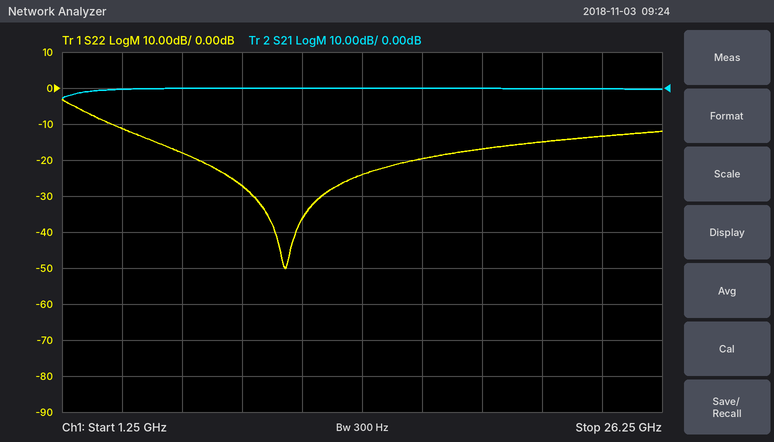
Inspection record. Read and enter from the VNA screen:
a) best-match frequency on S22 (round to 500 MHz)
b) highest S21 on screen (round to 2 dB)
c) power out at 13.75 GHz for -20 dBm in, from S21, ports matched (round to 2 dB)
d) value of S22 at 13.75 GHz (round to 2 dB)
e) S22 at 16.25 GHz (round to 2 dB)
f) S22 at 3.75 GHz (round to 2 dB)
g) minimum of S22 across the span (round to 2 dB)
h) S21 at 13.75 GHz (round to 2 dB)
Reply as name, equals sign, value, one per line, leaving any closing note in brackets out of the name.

best-match frequency on S22 = 10.5 GHz
highest S21 on screen = 0 dB
power out at 13.75 GHz for -20 dBm in, from S21, ports matched = -20 dBm
value of S22 at 13.75 GHz = -24 dB
S22 at 16.25 GHz = -20 dB
S22 at 3.75 GHz = -12 dB
minimum of S22 across the span = -50 dB
S21 at 13.75 GHz = 0 dB
